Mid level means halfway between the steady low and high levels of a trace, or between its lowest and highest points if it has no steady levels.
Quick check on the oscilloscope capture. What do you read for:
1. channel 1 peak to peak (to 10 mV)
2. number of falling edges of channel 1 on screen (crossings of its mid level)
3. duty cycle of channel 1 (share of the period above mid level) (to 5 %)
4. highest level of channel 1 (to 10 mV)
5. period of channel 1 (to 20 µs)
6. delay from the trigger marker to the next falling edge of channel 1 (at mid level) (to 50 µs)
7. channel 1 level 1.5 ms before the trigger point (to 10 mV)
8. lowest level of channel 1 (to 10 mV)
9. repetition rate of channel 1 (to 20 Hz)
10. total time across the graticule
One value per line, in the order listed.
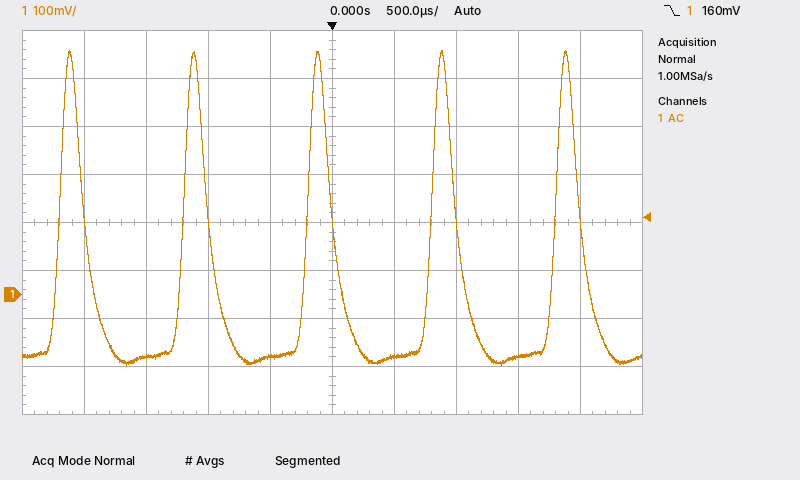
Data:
660 mV
5
20 %
510 mV
1.00 ms
1.00 ms
-130 mV
-150 mV
1.00 kHz
5 ms
